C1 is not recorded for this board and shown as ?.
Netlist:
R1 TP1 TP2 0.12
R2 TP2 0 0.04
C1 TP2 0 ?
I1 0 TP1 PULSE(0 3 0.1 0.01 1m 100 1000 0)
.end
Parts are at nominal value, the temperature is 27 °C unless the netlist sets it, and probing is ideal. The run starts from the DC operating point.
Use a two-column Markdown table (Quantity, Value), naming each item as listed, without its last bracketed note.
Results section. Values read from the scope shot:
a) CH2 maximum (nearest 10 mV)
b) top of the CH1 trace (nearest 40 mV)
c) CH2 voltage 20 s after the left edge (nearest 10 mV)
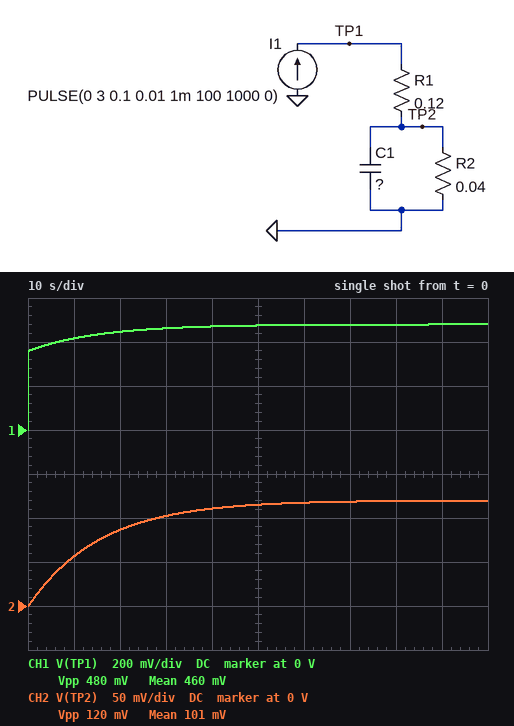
| Quantity | Value |
|---|---|
| CH2 maximum | 120 mV |
| top of the CH1 trace | 480 mV |
| CH2 voltage 20 s after the left edge | 90 mV |
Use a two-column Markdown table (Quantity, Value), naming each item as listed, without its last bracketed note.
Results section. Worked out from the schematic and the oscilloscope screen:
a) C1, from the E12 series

| Quantity | Value |
|---|---|
| C1, from the E12 series | 390 F |
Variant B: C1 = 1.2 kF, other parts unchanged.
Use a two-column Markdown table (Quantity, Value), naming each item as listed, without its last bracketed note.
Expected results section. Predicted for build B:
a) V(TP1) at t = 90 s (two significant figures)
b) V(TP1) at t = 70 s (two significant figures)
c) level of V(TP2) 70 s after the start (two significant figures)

| Quantity | Value |
|---|---|
| V(TP1) at t = 90 s | 460 mV |
| V(TP1) at t = 70 s | 450 mV |
| level of V(TP2) 70 s after the start | 92 mV |
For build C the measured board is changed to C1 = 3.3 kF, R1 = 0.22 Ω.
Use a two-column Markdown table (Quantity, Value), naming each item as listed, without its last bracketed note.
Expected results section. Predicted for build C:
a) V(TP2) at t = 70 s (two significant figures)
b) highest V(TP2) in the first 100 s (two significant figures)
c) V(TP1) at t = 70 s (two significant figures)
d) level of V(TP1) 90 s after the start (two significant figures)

| Quantity | Value |
|---|---|
| V(TP2) at t = 70 s | 49 mV |
| highest V(TP2) in the first 100 s | 64 mV |
| V(TP1) at t = 70 s | 710 mV |
| level of V(TP1) 90 s after the start | 720 mV |
